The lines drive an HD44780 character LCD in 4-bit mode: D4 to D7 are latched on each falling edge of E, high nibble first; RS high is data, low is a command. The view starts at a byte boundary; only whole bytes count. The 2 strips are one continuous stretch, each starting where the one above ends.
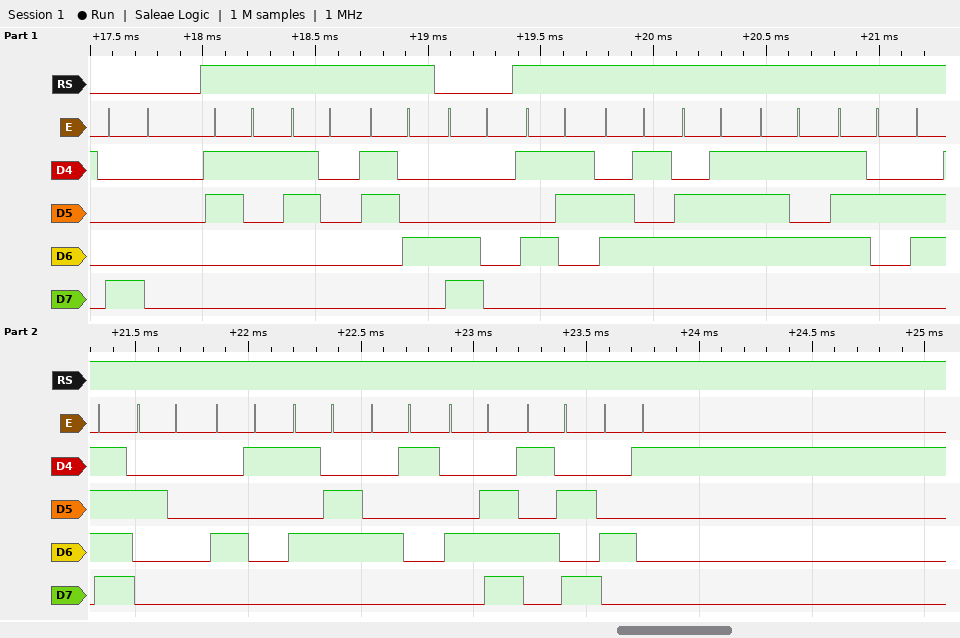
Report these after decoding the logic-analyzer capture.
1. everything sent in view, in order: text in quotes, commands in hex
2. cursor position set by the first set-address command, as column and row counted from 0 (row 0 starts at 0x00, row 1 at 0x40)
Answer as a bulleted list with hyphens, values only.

- 0x80 "104" 0xC0 "Seguro AVANZA"
- column 0, row 0
